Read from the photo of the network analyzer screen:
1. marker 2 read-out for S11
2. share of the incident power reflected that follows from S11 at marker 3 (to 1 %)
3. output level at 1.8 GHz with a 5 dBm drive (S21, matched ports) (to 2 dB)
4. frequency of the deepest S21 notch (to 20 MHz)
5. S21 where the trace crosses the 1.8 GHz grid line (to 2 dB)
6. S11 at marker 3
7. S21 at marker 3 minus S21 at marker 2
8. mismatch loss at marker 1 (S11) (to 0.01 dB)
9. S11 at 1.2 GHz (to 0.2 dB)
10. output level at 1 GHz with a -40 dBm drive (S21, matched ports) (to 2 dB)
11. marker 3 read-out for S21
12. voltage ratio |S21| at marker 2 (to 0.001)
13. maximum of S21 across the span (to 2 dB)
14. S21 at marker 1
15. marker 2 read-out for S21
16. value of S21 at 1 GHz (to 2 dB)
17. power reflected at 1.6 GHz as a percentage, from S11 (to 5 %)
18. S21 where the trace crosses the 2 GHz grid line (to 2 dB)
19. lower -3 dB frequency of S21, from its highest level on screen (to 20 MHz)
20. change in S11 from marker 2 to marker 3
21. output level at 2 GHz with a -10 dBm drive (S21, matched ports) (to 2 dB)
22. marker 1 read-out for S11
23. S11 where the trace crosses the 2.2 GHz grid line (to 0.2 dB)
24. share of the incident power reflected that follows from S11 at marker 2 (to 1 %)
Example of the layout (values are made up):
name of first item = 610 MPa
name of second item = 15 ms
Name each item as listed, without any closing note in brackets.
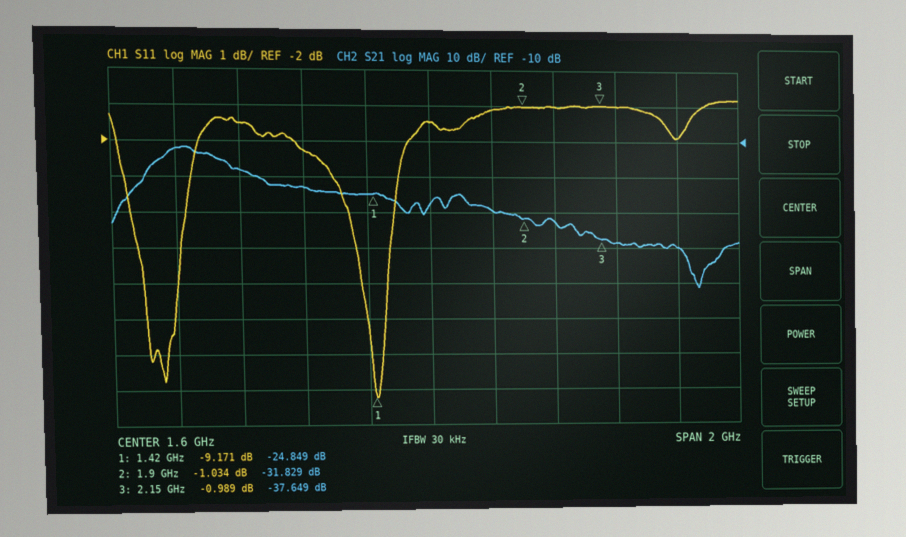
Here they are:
marker 2 read-out for S11 = -1.034 dB
share of the incident power reflected that follows from S11 at marker 3 = 80 %
output level at 1.8 GHz with a 5 dBm drive (S21, matched ports) = -24 dBm
frequency of the deepest S21 notch = 2.46 GHz
S21 where the trace crosses the 1.8 GHz grid line = -30 dB
S11 at marker 3 = -0.989 dB
S21 at marker 3 minus S21 at marker 2 = -5.820 dB
mismatch loss at marker 1 (S11) = 0.56 dB
S11 at 1.2 GHz = -2.2 dB
output level at 1 GHz with a -40 dBm drive (S21, matched ports) = -58 dBm
marker 3 read-out for S21 = -37.649 dB
voltage ratio |S21| at marker 2 = 0.026
maximum of S21 across the span = -12 dB
S21 at marker 1 = -24.849 dB
marker 2 read-out for S21 = -31.829 dB
value of S21 at 1 GHz = -18 dB
power reflected at 1.6 GHz as a percentage, from S11 = 70 %
S21 where the trace crosses the 2 GHz grid line = -32 dB
lower -3 dB frequency of S21, from its highest level on screen = 760 MHz
change in S11 from marker 2 to marker 3 = 0.045 dB
output level at 2 GHz with a -10 dBm drive (S21, matched ports) = -42 dBm
marker 1 read-out for S11 = -9.171 dB
S11 where the trace crosses the 2.2 GHz grid line = -1.0 dB
share of the incident power reflected that follows from S11 at marker 2 = 79 %
